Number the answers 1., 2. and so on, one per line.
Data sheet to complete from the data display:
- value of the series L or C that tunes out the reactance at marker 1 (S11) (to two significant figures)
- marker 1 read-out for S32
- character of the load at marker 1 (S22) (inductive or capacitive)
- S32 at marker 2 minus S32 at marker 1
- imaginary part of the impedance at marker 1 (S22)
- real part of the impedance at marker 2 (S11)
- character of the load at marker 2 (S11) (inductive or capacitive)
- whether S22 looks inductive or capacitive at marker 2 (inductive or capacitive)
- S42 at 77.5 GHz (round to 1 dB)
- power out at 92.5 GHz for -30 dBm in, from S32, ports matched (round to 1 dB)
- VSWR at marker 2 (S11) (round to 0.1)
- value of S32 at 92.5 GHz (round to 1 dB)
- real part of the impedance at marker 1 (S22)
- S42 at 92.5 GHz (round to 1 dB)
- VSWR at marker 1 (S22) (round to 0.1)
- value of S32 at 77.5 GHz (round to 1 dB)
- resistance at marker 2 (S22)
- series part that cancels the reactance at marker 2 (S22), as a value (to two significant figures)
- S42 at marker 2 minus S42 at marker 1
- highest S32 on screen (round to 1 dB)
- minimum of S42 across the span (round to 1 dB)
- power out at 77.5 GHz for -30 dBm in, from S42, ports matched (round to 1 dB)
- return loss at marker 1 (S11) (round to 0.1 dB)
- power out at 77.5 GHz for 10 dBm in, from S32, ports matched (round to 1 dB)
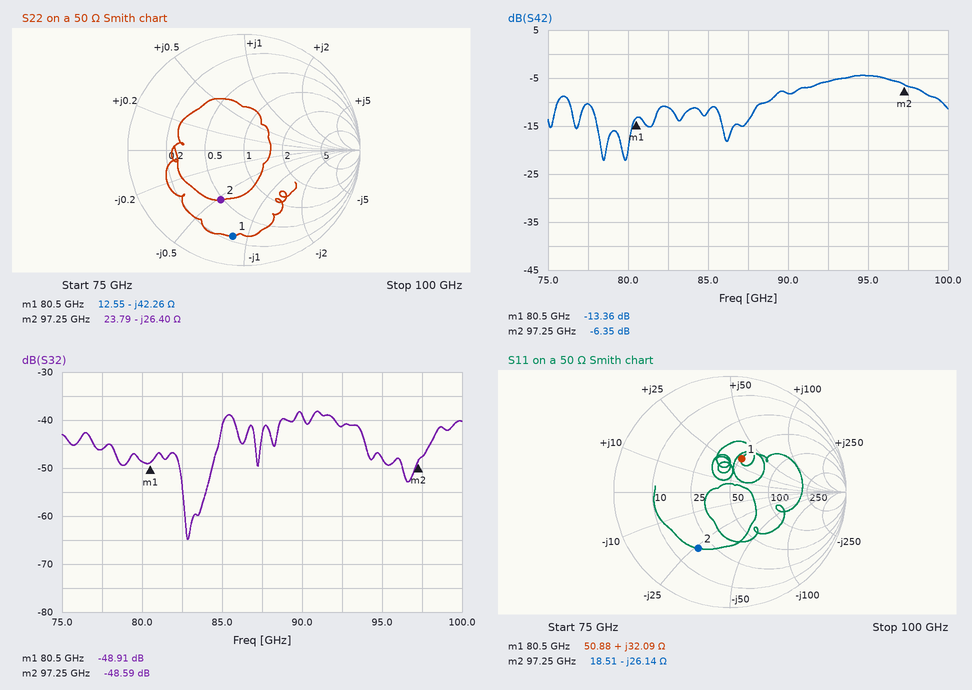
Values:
1. 62 fF
2. -48.91 dB
3. capacitive
4. 0.32 dB
5. -42.26 Ω
6. 18.51 Ω
7. capacitive
8. capacitive
9. -10 dB
10. -71 dBm
11. 3.5
12. -41 dB
13. 12.55 Ω
14. -6 dB
15. 6.9
16. -46 dB
17. 23.79 Ω
18. 43 pH
19. 7.01 dB
20. -38 dB
21. -22 dB
22. -40 dBm
23. 10.4 dB
24. -36 dBm
